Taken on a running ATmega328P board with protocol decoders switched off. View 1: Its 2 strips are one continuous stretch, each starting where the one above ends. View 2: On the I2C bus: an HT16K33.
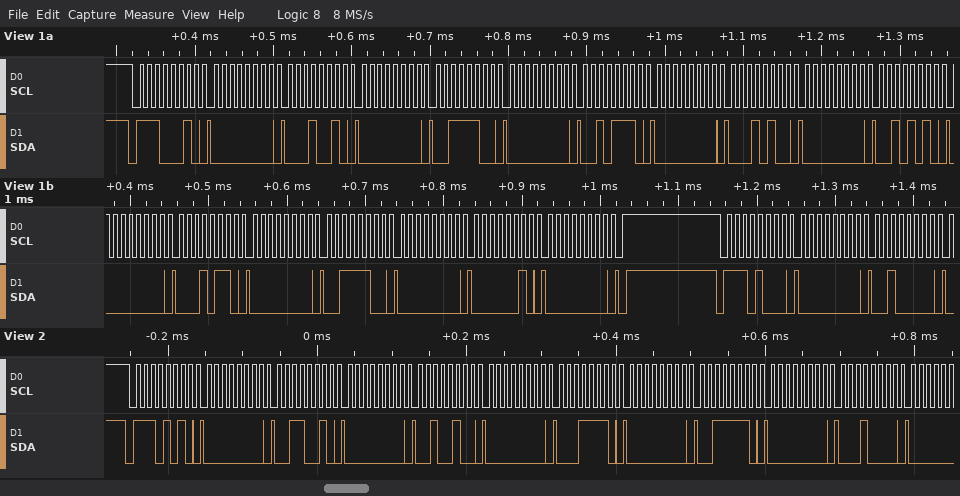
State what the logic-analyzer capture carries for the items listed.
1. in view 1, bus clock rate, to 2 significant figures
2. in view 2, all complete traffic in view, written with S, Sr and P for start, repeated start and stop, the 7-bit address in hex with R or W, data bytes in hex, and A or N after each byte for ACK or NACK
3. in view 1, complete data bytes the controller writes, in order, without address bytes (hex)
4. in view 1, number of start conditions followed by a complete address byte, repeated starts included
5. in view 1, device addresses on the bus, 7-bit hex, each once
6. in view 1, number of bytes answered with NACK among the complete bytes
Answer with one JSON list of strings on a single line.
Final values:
["100 kHz", "S 75W A 00 A 32 A 00 A 24 A 00 A 1E A 00 A 3E A 00 A 10 A", "00 12 00 3C 00 2E 00 14 00 2A 00 16 00 3C 00 02 00 00 20", "2", "0x71 0x74", "0"]
